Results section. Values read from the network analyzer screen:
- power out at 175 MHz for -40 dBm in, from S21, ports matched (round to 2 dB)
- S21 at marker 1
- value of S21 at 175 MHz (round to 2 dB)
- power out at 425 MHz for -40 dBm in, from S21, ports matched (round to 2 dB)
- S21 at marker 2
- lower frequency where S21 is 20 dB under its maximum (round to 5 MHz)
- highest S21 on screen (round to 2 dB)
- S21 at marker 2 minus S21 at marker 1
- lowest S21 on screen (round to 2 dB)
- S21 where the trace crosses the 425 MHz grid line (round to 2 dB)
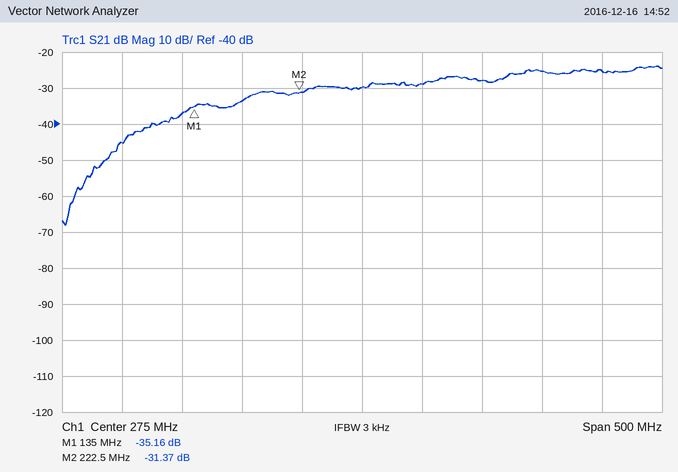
-74 dBm
-35.16 dB
-34 dB
-66 dBm
-31.37 dB
80 MHz
-24 dB
3.79 dB
-68 dB
-26 dB
